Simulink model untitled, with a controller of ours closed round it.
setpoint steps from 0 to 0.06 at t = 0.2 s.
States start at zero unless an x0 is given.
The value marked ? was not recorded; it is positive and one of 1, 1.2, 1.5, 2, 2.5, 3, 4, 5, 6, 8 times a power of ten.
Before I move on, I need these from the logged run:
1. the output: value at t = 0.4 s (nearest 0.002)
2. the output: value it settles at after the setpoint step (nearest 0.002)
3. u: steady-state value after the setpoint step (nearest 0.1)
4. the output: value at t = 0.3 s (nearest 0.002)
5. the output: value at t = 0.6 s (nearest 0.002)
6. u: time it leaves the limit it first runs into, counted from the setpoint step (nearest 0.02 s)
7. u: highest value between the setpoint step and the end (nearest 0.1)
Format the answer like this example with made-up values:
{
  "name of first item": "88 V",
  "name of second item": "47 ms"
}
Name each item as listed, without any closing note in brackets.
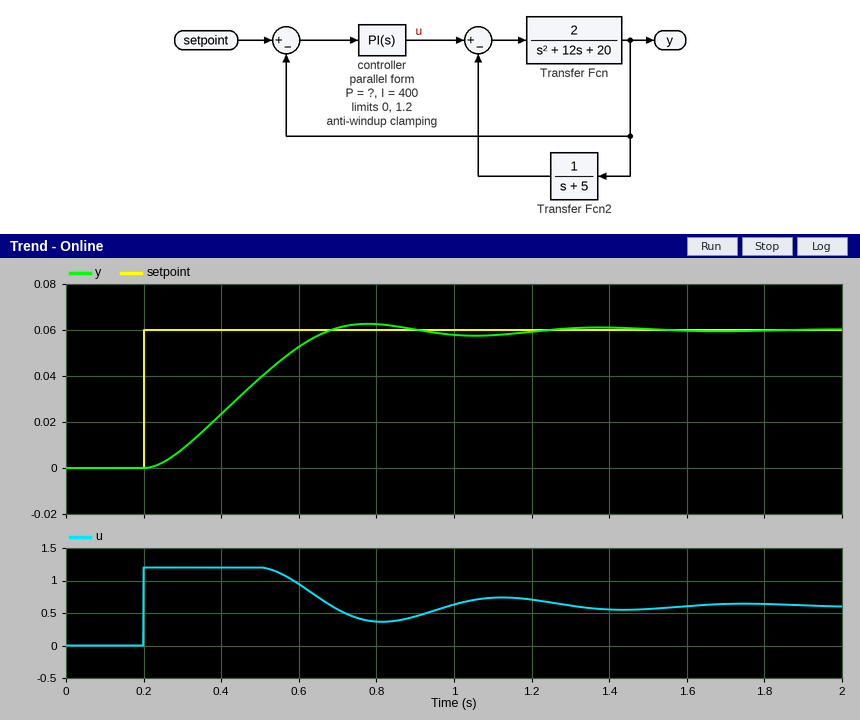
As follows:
{
  "the output: value at t = 0.4 s": "0.024",
  "the output: value it settles at after the setpoint step": "0.060",
  "u: steady-state value after the setpoint step": "0.6",
  "the output: value at t = 0.3 s": "0.008",
  "the output: value at t = 0.6 s": "0.052",
  "u: time it leaves the limit it first runs into, counted from the setpoint step": "0.32 s",
  "u: highest value between the setpoint step and the end": "1.2"
}
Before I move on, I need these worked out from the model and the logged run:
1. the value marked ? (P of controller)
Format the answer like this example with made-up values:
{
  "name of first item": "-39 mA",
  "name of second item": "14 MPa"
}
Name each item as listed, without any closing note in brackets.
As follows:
{
  "the value marked ?": "60"
}
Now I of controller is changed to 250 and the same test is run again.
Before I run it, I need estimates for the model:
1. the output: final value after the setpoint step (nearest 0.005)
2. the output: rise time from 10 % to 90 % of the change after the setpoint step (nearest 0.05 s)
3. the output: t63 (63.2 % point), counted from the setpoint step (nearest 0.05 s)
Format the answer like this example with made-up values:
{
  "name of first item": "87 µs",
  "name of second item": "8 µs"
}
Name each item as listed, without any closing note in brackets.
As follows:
{
  "the output: final value after the setpoint step": "0.060",
  "the output: rise time from 10 % to 90 % of the change after the setpoint step": "0.35 s",
  "the output: t63 (63.2 % point), counted from the setpoint step": "0.30 s"
}
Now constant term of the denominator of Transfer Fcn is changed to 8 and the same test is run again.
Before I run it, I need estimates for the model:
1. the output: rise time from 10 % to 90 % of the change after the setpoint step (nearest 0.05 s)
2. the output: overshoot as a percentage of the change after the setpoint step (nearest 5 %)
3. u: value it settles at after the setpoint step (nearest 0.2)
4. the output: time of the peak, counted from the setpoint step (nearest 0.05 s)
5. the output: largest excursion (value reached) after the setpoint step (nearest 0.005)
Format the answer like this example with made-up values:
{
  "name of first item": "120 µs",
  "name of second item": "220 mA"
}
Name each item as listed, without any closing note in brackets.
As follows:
{
  "the output: rise time from 10 % to 90 % of the change after the setpoint step": "0.30 s",
  "the output: overshoot as a percentage of the change after the setpoint step": "10 %",
  "u: value it settles at after the setpoint step": "0.2",
  "the output: time of the peak, counted from the setpoint step": "0.55 s",
  "the output: largest excursion (value reached) after the setpoint step": "0.065"
}
